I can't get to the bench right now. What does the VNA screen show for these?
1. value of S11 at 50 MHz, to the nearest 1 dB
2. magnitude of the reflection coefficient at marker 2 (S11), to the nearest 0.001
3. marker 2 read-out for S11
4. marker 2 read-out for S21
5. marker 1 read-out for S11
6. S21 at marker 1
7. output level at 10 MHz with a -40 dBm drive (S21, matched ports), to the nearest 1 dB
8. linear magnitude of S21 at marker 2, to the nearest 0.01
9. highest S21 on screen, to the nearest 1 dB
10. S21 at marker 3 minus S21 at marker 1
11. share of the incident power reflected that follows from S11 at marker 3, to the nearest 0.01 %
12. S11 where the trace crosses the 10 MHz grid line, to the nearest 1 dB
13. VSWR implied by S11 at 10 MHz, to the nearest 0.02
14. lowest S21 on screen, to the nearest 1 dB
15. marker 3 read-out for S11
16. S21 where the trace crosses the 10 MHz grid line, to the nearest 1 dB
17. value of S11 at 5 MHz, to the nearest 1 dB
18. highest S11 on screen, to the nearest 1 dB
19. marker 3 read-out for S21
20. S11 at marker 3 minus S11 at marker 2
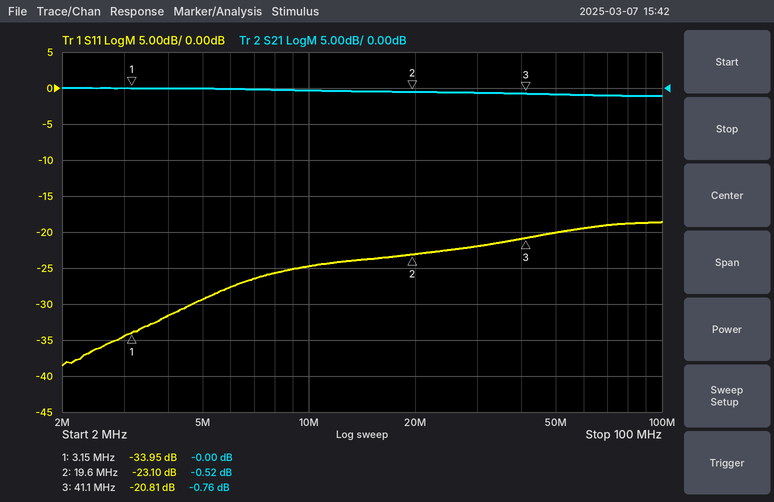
-20 dB
0.070
-23.10 dB
-0.52 dB
-33.95 dB
-0.00 dB
-40 dBm
0.94
0 dB
-0.76 dB
0.83 %
-25 dB
1.12
-1 dB
-20.81 dB
0 dB
-29 dB
-19 dB
-0.76 dB
2.29 dB
